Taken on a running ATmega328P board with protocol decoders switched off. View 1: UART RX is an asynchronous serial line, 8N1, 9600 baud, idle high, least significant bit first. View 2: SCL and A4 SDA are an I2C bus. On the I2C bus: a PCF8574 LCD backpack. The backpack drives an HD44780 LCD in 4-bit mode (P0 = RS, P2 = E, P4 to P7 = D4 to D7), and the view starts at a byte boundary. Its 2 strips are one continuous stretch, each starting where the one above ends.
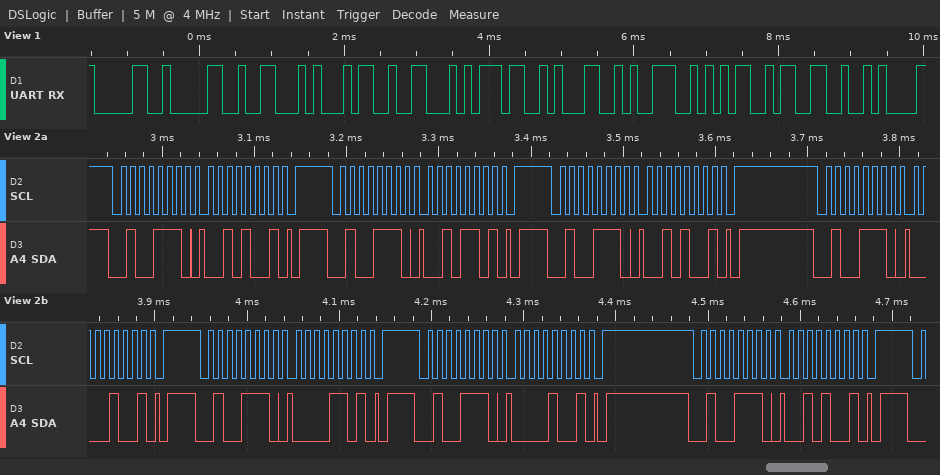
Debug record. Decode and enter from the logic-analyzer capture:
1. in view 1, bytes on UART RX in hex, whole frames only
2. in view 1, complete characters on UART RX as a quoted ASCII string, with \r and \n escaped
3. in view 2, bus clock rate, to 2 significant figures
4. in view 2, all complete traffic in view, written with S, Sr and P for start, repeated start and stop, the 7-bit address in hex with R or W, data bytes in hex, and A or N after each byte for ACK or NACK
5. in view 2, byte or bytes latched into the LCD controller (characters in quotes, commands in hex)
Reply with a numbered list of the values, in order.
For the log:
1. 0x30 0x30 0x46 0x34 0x46 0x37 0x31 0x39 0x35 0x33 0x0A
2. "00F4F71953\n"
3. 100 kHz
4. S 27W A 29 A P S 27W A 2D A P S 27W A 29 A P S 27W A 09 A P S 27W A 0D A P S 27W A 09 A P S 27W A 29 A P
5. ' '
